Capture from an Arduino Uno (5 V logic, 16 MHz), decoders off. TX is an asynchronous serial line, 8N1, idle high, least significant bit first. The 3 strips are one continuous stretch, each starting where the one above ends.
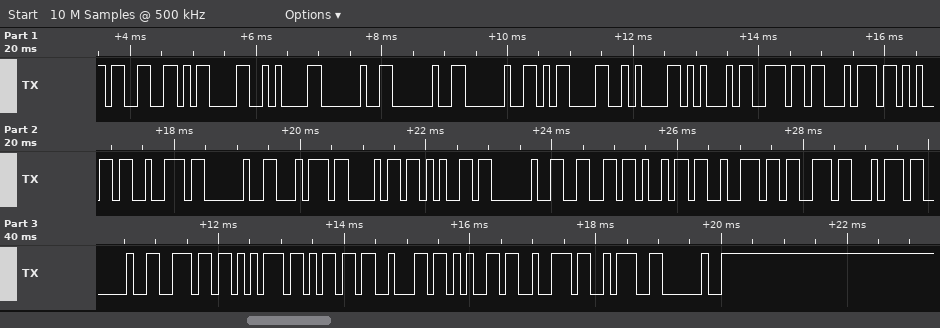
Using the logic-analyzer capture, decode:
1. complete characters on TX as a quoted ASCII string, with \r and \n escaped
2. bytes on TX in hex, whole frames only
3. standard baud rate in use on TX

"3\r\n   \r\nEnter the first number: "
33 0D 0A 20 20 20 0D 0A 45 6E 74 65 72 20 74 68 65 20 66 69 72 73 74 20 6E 75 6D 62 65 72 3A 20
9600 baud
